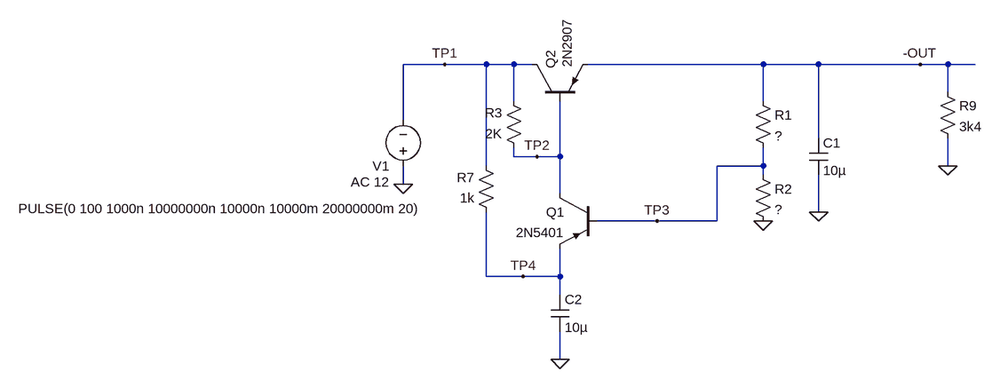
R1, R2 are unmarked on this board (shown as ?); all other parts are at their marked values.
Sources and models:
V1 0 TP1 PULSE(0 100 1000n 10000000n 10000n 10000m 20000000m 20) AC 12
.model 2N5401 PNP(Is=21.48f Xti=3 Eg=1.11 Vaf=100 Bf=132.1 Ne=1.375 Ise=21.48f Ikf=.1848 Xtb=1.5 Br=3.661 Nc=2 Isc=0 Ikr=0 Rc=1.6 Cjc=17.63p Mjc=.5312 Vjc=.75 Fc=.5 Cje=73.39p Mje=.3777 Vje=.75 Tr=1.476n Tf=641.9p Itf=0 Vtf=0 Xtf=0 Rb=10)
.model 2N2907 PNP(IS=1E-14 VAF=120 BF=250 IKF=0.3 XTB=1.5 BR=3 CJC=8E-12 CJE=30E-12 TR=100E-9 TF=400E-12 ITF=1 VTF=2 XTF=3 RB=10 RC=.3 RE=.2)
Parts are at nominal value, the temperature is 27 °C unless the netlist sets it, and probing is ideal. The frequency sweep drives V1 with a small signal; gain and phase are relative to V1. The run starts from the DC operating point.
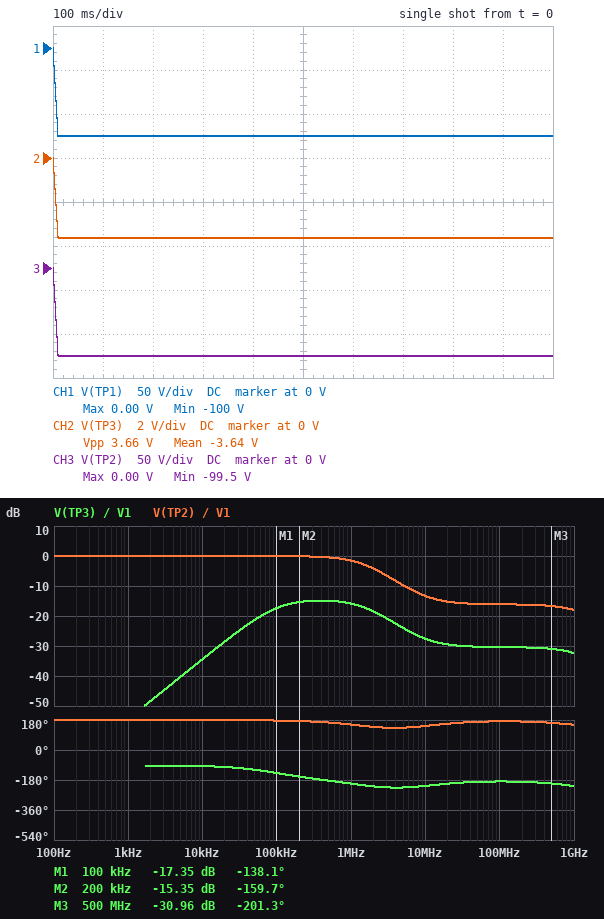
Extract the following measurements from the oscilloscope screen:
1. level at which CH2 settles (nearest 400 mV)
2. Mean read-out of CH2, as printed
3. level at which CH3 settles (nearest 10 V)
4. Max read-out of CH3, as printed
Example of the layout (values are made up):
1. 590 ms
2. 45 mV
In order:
1. -3.6 V
2. -3.64 V
3. -100 V
4. 0.00 V
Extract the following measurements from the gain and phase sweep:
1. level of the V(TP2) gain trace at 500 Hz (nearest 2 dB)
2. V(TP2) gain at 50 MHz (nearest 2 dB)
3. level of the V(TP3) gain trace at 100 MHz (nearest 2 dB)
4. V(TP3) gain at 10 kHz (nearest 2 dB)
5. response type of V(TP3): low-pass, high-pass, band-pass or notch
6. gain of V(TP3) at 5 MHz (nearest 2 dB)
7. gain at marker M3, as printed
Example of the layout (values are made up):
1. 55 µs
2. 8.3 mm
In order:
1. 0 dB
2. -16 dB
3. -30 dB
4. -34 dB
5. band-pass
6. -24 dB
7. -30.96 dB
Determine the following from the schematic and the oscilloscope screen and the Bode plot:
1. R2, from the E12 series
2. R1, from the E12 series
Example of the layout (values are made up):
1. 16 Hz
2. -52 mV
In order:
1. 18 kΩ
2. 470 kΩ
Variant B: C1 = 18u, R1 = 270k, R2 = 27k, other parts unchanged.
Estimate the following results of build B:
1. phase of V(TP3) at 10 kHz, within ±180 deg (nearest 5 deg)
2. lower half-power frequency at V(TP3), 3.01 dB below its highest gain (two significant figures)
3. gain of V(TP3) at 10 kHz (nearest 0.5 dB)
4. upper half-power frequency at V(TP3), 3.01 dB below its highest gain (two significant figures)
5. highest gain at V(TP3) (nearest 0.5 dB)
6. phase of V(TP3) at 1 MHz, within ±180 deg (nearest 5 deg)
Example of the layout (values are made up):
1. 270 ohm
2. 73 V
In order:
1. -100 deg
2. 65 kHz
3. -31.5 dB
4. 1.7 MHz
5. -14.5 dB
6. 155 deg
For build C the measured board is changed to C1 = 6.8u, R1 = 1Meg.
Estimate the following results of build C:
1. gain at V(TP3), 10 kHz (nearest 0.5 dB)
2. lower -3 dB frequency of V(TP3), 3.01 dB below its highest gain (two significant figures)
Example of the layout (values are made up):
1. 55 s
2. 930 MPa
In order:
1. -34.0 dB
2. 88 kHz
